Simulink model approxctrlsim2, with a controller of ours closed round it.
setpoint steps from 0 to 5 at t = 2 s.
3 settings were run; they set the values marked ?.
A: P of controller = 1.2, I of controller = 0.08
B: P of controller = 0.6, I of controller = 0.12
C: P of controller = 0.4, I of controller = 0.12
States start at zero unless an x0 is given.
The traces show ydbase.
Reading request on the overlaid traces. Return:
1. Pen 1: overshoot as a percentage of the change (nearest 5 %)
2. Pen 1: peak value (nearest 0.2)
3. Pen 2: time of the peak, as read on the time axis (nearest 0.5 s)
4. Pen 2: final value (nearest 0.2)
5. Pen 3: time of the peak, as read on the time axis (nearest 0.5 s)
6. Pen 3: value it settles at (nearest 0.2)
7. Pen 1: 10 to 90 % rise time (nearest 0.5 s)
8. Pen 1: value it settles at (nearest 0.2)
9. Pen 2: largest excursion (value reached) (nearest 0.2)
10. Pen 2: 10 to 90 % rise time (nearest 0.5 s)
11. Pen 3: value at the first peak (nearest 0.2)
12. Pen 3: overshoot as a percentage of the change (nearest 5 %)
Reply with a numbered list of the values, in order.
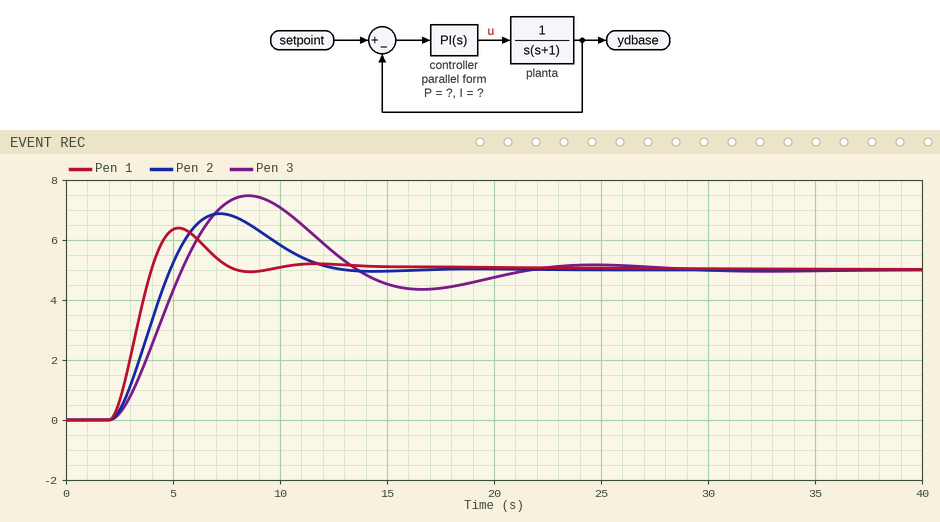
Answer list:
1. 30 %
2. 6.4
3. 7.0 s
4. 5.0
5. 8.5 s
6. 5.0
7. 1.5 s
8. 5.0
9. 6.8
10. 2.0 s
11. 7.4
12. 50 %
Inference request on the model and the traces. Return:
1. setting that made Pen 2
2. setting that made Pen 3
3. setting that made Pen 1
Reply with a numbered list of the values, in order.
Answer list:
1. B
2. C
3. A
